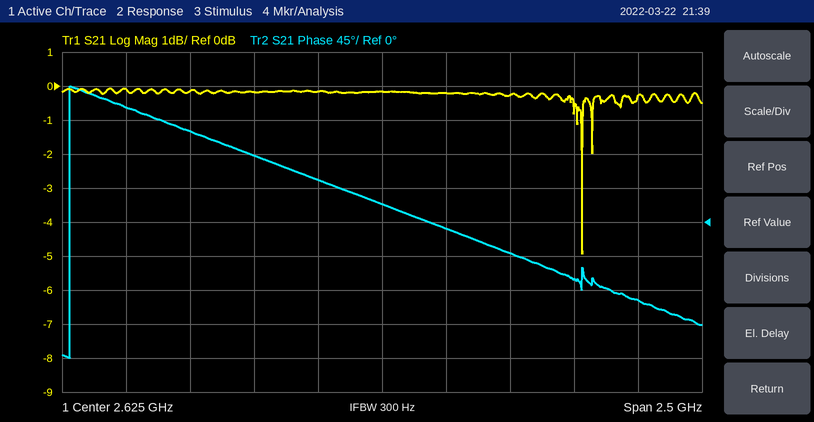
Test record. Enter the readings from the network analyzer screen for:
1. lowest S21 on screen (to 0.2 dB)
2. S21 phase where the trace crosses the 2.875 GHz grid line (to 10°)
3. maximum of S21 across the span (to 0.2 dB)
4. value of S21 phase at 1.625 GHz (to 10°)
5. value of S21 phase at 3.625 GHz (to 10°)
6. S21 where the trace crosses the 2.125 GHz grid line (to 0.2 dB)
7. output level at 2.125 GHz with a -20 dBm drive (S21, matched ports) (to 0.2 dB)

-5.0 dB
-10°
0.0 dB
150°
-100°
-0.2 dB
-20.2 dBm
